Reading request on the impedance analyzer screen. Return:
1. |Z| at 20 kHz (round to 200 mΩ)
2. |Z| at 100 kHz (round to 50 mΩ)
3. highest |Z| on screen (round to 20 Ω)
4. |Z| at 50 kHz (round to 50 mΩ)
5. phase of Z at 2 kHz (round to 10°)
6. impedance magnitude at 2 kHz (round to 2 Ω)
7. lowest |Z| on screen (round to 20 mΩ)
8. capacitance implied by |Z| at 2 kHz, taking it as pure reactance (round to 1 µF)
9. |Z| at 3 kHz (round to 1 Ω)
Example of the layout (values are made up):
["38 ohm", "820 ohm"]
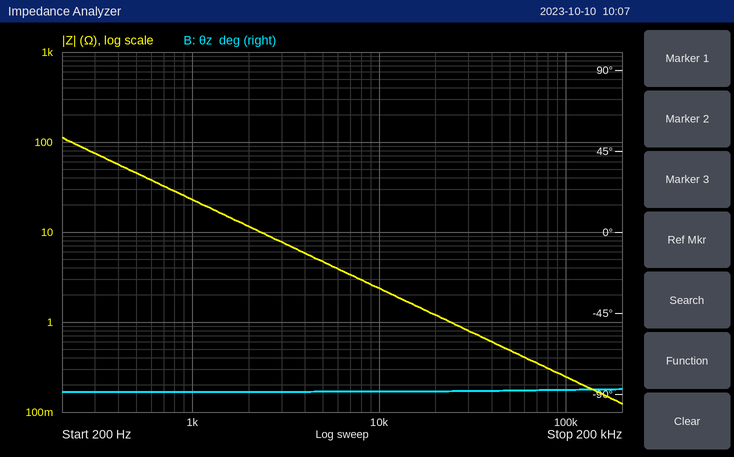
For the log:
["1.2 Ω", "250 mΩ", "120 Ω", "500 mΩ", "-90°", "12 Ω", "120 mΩ", "7 µF", "8 Ω"]
